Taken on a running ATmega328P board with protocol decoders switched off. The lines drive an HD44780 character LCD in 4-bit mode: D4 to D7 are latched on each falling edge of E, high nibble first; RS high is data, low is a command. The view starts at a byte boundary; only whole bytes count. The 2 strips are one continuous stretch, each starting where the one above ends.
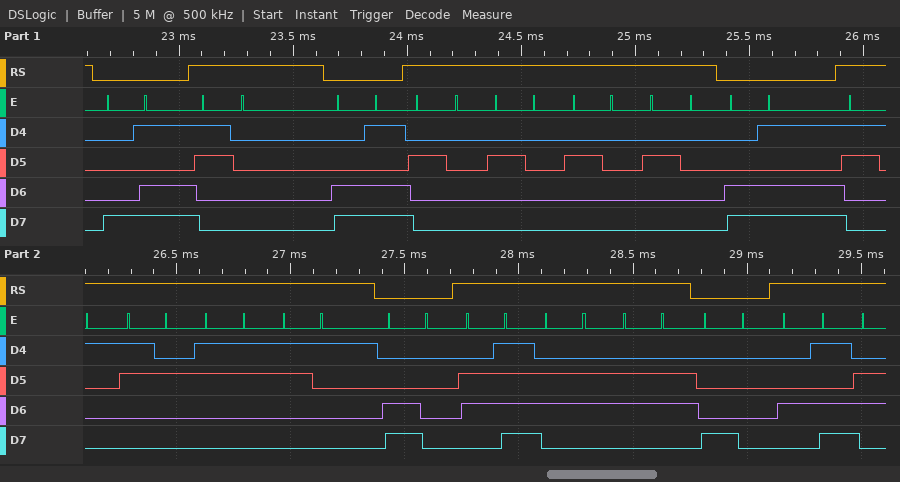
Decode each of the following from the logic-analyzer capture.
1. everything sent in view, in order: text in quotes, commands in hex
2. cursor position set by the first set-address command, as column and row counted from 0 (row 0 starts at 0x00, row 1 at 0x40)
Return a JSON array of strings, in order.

["0x8D \"0\" 0xCD \"    \" 0xCD \"1231\" 0xC0 \"off\" 0x80 \"M\"", "column 13, row 0"]
